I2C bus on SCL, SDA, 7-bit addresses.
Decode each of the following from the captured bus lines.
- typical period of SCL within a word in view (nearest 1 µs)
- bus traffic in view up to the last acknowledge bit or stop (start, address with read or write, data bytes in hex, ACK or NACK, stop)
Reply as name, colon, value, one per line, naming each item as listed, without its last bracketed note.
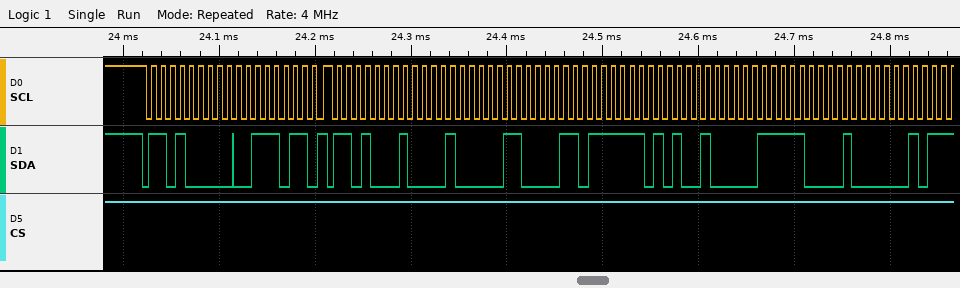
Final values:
typical period of SCL within a word in view: 10 µs
bus traffic in view up to the last acknowledge bit or stop: start, address 68 write ACK, 3B ACK, repeated start, address 68 read ACK, 10 ACK, C3 ACK, FD ACK, 90 ACK, F8 ACK, 81 ACK
